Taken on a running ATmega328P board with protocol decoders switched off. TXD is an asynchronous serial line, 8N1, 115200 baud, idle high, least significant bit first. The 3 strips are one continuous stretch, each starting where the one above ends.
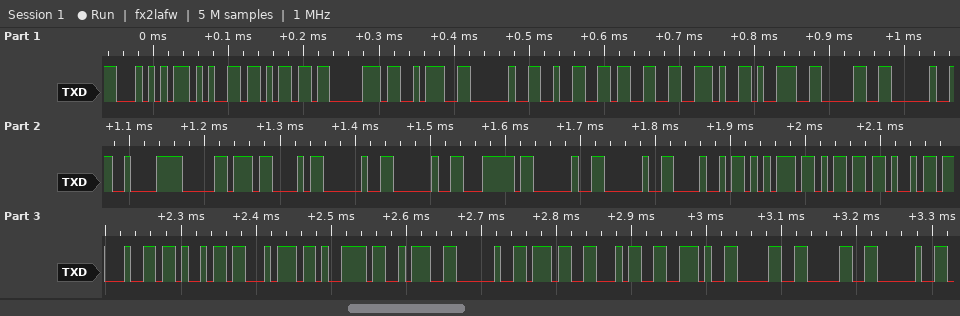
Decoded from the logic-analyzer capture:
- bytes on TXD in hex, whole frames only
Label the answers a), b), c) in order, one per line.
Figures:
a) 0x54 0x65 0x6D 0x70 0x3A 0x20 0x32 0x33 0x2E 0x39 0x30 0x20 0xC2 0xB0 0x43 0x20 0x20 0x7C 0x20 0x20 0x48 0x75 0x6D 0x69 0x64 0x69 0x74 0x79 0x3A 0x20 0x37 0x34 0x2E 0x30 0x30 0x20
